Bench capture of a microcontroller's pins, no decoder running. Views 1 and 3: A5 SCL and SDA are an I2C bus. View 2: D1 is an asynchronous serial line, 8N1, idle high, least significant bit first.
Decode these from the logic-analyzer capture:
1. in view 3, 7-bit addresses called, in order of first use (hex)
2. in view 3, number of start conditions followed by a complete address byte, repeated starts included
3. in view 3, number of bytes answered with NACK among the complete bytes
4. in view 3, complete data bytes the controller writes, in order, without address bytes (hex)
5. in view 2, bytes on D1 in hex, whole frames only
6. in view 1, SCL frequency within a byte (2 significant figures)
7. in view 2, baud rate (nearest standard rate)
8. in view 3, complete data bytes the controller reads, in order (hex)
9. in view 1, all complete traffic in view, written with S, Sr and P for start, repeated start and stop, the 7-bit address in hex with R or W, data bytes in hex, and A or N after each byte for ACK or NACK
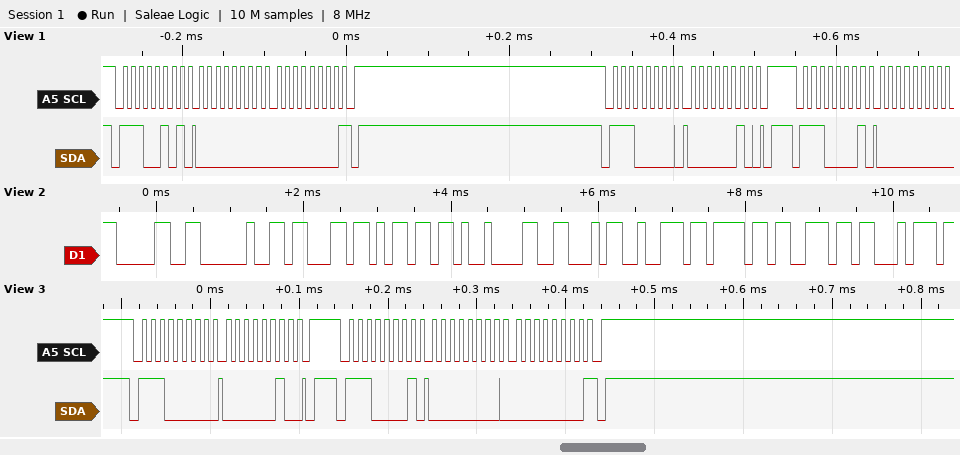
0x70
2
1
02
0x30 0x20 0x63 0x6D 0x09 0x46 0x72 0x6F 0x6E 0x74
100 kHz
9600 baud
00 00
S 72R A 00 A 00 N P S 70W A 02 A P S 70R A 00 A
